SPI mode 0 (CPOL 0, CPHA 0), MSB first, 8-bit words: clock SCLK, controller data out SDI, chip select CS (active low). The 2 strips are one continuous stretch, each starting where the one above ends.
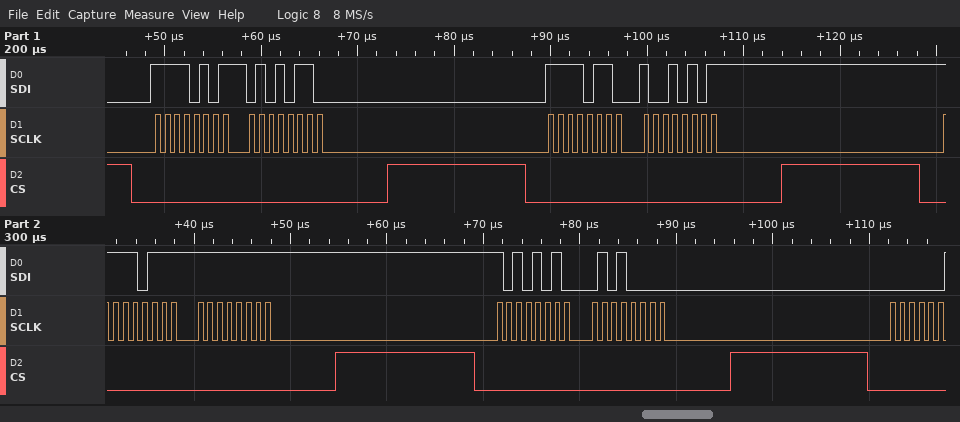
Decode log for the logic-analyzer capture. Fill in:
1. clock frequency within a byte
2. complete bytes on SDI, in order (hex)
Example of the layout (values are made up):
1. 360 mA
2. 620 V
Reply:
1. 1 MHz
2. F5 56 F6 95 F7 FF AA 50
